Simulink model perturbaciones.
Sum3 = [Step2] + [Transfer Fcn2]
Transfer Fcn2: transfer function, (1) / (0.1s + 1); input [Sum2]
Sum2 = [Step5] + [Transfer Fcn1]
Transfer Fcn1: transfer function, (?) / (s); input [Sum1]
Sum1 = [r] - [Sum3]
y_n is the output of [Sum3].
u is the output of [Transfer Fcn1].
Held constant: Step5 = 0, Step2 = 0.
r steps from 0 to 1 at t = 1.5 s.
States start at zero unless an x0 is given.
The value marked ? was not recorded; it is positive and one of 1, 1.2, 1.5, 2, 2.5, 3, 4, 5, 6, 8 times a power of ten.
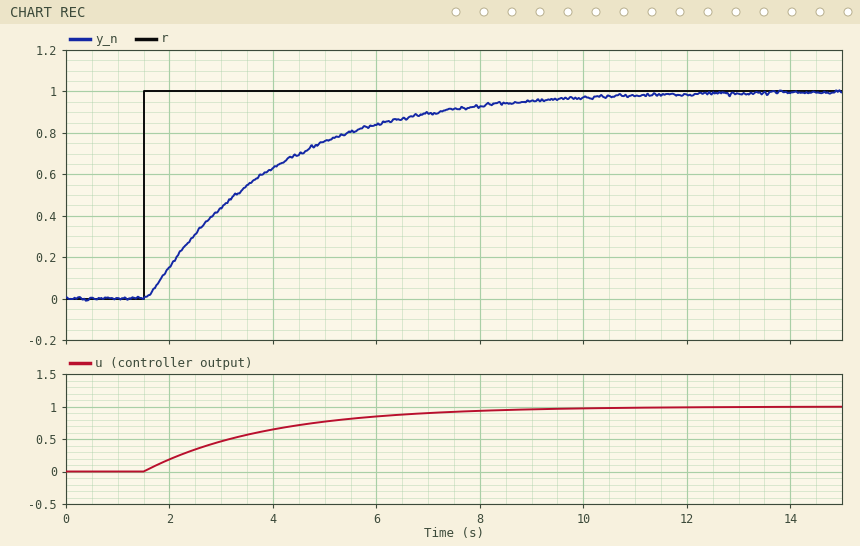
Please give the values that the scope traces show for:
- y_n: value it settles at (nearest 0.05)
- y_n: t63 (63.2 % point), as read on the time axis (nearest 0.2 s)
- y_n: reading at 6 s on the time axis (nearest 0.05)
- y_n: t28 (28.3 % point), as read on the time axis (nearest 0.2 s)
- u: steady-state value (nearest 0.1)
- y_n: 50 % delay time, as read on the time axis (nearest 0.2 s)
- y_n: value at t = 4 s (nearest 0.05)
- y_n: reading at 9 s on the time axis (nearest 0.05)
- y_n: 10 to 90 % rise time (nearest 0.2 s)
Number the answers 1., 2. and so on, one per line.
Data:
1. 1.00
2. 4.0 s
3. 0.85
4. 2.4 s
5. 1.0
6. 3.2 s
7. 0.65
8. 0.95
9. 5.2 s
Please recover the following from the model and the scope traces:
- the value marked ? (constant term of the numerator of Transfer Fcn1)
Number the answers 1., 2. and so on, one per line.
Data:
1. 0.4
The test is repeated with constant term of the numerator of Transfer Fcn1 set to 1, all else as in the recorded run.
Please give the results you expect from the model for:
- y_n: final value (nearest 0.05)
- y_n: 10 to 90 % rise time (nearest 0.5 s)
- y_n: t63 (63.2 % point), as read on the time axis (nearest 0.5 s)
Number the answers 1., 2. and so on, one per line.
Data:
1. 1.00
2. 2.0 s
3. 2.5 s
